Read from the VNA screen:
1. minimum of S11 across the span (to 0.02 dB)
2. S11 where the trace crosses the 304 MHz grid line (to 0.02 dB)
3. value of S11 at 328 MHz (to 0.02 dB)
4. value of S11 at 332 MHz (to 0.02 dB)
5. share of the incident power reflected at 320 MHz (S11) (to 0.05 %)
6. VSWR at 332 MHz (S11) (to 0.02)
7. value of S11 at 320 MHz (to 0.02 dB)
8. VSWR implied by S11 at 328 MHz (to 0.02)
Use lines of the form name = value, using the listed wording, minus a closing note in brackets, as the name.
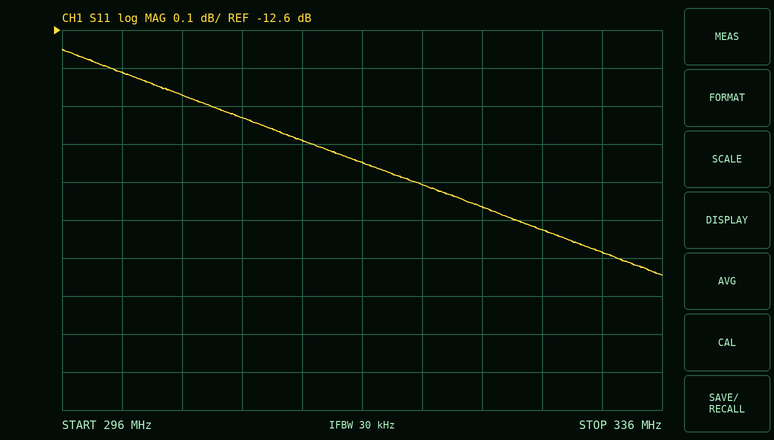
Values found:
minimum of S11 across the span = -13.24 dB
S11 where the trace crosses the 304 MHz grid line = -12.78 dB
value of S11 at 328 MHz = -13.12 dB
value of S11 at 332 MHz = -13.18 dB
share of the incident power reflected at 320 MHz (S11) = 5.00 %
VSWR at 332 MHz (S11) = 1.56
value of S11 at 320 MHz = -13.00 dB
VSWR implied by S11 at 328 MHz = 1.56
